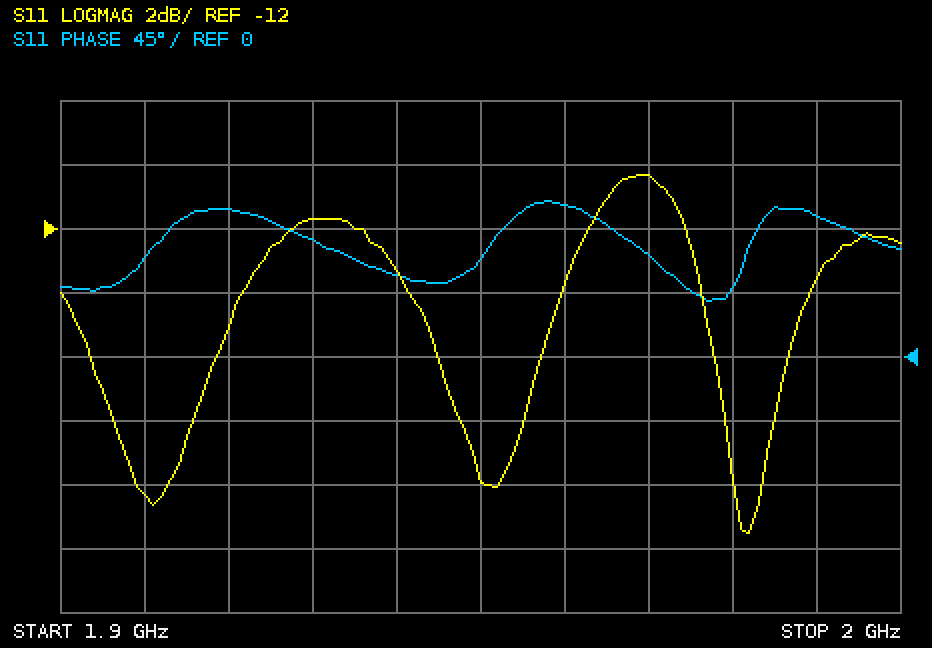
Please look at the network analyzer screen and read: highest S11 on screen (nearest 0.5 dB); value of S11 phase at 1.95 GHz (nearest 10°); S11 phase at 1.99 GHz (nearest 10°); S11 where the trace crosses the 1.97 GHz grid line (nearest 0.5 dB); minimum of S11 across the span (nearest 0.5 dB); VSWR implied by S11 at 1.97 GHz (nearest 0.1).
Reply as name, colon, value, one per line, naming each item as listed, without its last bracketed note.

highest S11 on screen: -10.5 dB
value of S11 phase at 1.95 GHz: 70°
S11 phase at 1.99 GHz: 100°
S11 where the trace crosses the 1.97 GHz grid line: -10.5 dB
minimum of S11 across the span: -21.5 dB
VSWR implied by S11 at 1.97 GHz: 1.9
